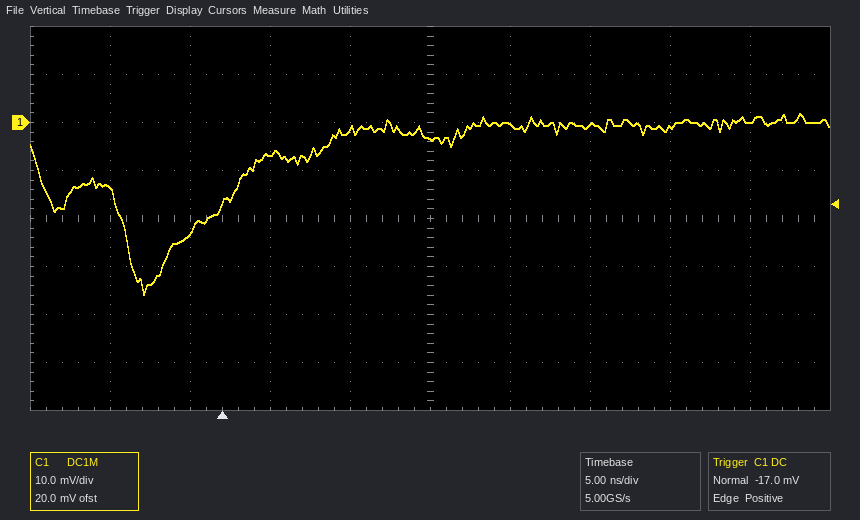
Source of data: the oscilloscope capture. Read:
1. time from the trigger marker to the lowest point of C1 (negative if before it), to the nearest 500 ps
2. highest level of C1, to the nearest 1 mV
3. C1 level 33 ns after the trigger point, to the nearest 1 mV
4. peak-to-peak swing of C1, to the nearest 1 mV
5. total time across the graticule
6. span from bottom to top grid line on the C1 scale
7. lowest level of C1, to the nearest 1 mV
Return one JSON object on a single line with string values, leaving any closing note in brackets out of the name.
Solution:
{"time from the trigger marker to the lowest point of C1 (negative if before it), to the nearest 500 ps": "-5.0 ns", "highest level of C1, to the nearest 1 mV": "2 mV", "C1 level 33 ns after the trigger point, to the nearest 1 mV": "0 mV", "peak-to-peak swing of C1, to the nearest 1 mV": "38 mV", "total time across the graticule": "50 ns", "span from bottom to top grid line on the C1 scale": "80 mV", "lowest level of C1, to the nearest 1 mV": "-36 mV"}
